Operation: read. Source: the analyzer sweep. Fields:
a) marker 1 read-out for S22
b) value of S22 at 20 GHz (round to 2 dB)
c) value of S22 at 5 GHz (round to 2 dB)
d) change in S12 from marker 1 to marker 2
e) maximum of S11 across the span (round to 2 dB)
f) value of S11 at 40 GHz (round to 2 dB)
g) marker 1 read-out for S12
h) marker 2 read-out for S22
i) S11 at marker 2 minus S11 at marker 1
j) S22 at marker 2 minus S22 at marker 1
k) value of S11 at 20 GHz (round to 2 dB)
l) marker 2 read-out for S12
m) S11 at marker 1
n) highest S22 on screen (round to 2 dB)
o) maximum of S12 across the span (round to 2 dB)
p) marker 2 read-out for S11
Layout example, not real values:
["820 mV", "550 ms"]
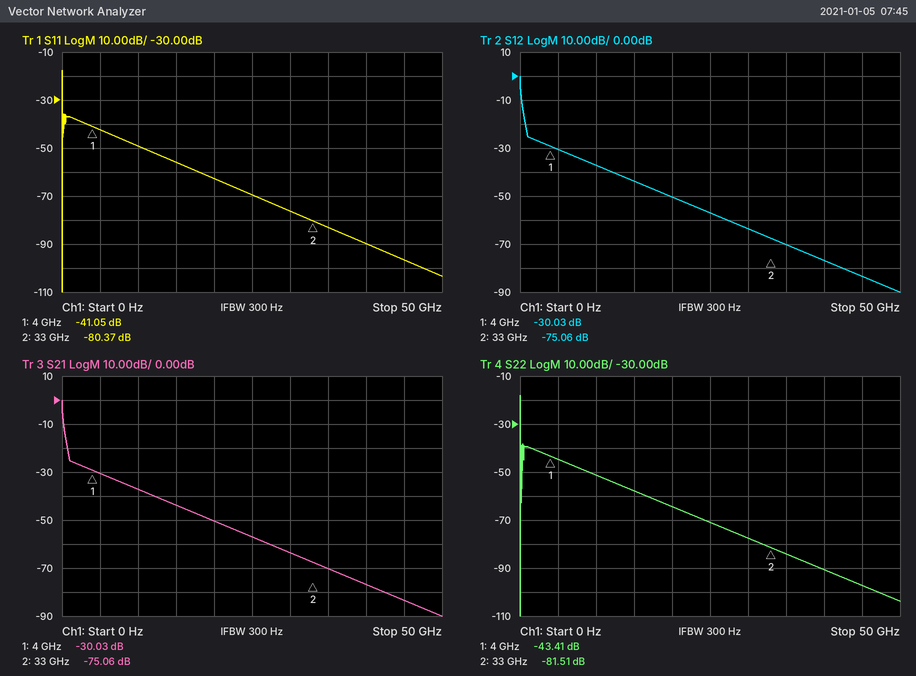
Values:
["-43.41 dB", "-64 dB", "-44 dB", "-45.03 dB", "-18 dB", "-90 dB", "-30.03 dB", "-81.51 dB", "-39.32 dB", "-38.10 dB", "-62 dB", "-75.06 dB", "-41.05 dB", "-18 dB", "0 dB", "-80.37 dB"]
